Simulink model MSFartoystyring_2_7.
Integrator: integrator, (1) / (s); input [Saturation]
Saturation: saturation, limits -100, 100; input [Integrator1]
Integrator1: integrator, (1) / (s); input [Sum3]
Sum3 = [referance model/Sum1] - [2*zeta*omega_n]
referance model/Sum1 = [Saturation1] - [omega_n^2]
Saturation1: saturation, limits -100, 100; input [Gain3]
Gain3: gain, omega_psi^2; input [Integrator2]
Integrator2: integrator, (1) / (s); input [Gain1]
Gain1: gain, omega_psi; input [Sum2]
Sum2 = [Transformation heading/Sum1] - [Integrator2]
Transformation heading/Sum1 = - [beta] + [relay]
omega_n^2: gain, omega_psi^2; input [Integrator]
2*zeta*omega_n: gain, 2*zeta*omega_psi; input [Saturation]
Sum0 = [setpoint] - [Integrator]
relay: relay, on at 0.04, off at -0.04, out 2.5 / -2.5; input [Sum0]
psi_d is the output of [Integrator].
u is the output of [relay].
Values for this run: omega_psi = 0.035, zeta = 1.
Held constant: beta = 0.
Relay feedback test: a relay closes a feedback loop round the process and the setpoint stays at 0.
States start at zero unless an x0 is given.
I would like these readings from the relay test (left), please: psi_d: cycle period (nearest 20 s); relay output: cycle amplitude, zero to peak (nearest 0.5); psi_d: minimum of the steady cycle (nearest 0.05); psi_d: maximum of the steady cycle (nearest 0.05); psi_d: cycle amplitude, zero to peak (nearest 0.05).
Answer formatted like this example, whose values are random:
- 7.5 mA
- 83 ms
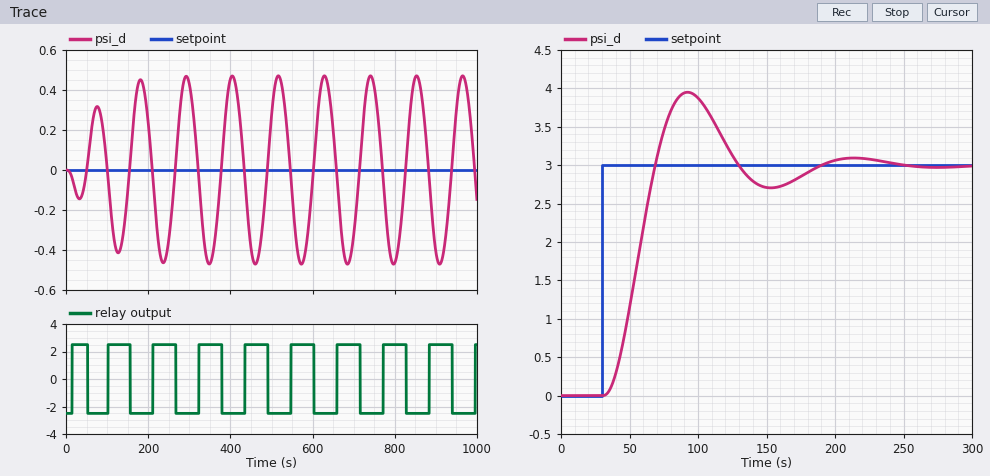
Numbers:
- 120 s
- 2.5
- -0.45
- 0.45
- 0.45
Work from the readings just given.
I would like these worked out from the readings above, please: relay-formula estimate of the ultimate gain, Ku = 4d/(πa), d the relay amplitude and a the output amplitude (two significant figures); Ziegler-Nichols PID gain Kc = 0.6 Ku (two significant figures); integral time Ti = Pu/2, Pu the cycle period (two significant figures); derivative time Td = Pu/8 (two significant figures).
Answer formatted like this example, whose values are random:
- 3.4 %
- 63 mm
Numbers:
- 7.1
- 4.3
- 60 s
- 15 s
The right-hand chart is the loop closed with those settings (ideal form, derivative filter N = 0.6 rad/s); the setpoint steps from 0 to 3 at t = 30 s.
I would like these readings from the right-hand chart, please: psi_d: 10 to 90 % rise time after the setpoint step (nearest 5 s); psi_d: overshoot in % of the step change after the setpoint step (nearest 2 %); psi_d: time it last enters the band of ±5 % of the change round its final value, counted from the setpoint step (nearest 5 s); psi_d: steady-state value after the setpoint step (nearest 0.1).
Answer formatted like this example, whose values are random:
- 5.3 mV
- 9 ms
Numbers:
- 25 s
- 32 %
- 145 s
- 3.0
